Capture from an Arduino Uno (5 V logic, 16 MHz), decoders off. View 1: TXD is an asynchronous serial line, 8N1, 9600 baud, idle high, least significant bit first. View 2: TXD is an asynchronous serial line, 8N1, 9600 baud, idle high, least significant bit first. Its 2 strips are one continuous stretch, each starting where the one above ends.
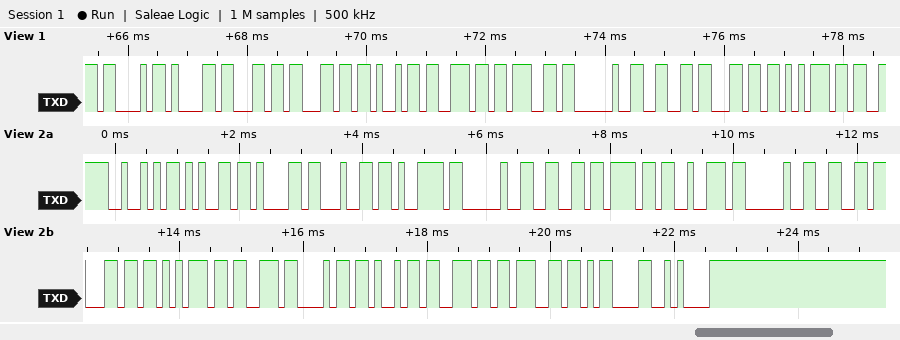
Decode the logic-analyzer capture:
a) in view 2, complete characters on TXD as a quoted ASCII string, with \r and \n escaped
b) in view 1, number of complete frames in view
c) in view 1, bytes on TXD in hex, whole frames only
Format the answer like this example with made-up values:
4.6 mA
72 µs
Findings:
"Ready for flushing\r\n"
11
0x43 0x61 0x6C 0x6C 0x69 0x6E 0x67 0x20 0x66 0x6C 0x75
